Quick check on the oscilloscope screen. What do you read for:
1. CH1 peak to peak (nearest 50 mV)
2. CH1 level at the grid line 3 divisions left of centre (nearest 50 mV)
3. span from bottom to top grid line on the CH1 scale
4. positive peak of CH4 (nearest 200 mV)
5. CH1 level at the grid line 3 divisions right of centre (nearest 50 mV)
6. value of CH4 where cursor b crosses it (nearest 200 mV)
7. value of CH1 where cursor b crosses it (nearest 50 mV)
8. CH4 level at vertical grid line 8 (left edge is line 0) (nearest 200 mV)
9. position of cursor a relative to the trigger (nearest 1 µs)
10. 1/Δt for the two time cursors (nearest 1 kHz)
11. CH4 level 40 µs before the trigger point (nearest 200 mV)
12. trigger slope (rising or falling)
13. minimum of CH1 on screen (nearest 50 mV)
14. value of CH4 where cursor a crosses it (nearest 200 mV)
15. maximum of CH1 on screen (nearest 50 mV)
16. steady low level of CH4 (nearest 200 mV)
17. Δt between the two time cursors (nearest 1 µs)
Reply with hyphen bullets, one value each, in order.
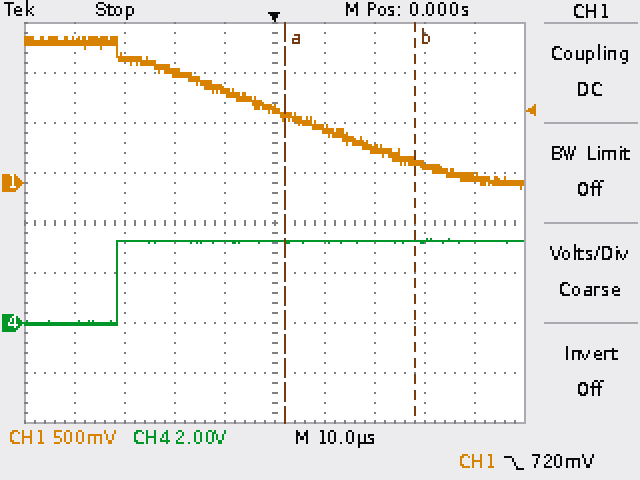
- 1.50 V
- 1.25 V
- 4 V
- 3.4 V
- 200 mV
- 3.2 V
- 200 mV
- 3.2 V
- +2 µs
- 38 kHz
- 0.0 V
- falling
- -50 mV
- 3.2 V
- 1.45 V
- 0.0 V
- 26 µs
